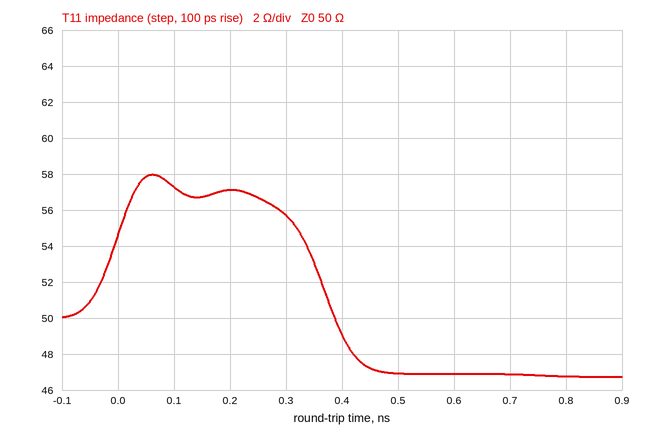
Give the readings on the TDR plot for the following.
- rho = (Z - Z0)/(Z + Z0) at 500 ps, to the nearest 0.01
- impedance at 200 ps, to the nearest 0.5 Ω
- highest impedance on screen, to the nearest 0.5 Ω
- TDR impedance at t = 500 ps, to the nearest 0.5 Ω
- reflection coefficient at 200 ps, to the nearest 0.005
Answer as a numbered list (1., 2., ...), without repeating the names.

1. -0.03
2. 57.0 Ω
3. 58.0 Ω
4. 47.0 Ω
5. +0.065
